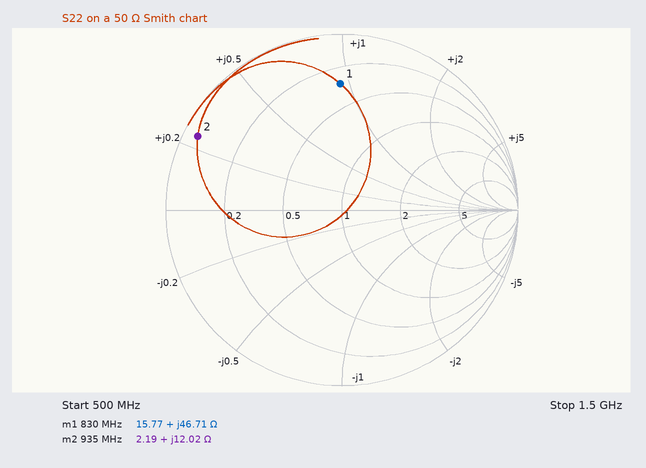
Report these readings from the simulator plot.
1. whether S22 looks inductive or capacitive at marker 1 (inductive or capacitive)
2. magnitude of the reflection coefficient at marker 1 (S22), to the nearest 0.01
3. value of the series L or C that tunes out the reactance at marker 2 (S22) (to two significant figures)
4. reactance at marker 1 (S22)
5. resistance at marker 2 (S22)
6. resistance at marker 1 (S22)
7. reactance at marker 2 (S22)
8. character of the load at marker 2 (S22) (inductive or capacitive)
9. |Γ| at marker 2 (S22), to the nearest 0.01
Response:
inductive
0.72
14 pF
+46.71 Ω
2.19 Ω
15.77 Ω
+12.02 Ω
inductive
0.92
